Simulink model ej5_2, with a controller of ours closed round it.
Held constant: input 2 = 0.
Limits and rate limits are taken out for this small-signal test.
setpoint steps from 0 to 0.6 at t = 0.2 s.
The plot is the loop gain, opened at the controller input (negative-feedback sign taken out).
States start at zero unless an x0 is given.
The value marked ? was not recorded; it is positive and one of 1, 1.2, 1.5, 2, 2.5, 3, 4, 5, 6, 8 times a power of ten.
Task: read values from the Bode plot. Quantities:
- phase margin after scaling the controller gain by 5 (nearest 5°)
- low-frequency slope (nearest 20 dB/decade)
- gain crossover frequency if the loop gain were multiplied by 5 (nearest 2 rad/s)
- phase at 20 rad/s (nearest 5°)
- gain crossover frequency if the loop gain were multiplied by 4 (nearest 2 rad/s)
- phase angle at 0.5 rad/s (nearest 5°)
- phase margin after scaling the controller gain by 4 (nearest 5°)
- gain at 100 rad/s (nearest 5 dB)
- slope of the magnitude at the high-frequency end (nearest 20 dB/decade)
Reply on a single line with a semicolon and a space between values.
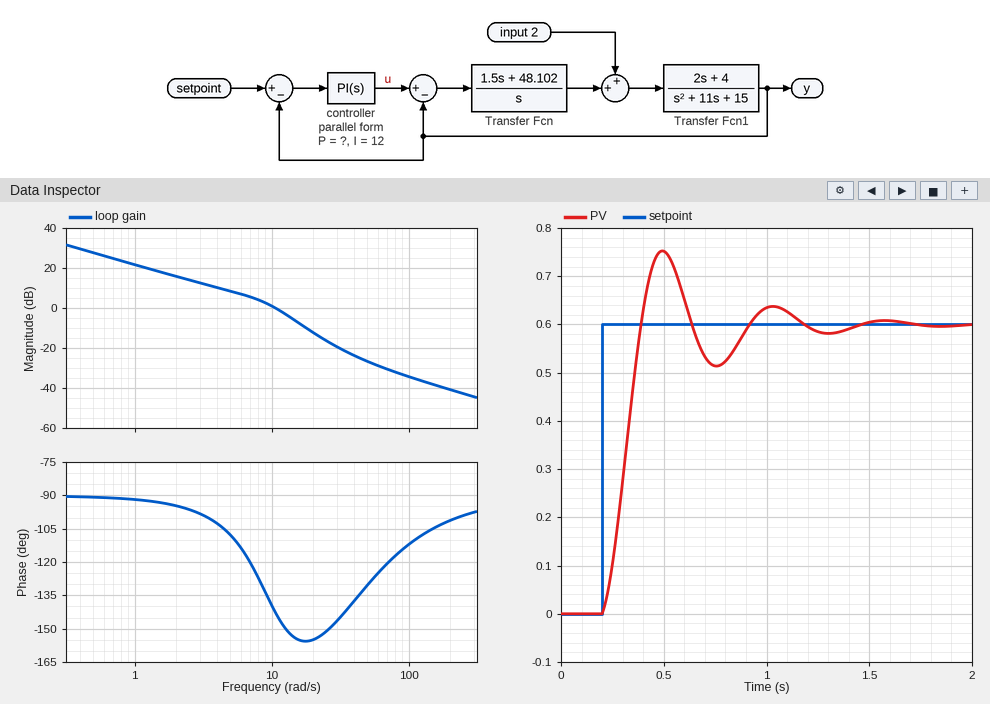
25°; -20 dB/decade; 22 rad/s; -155°; 20 rad/s; -90°; 25°; -35 dB; -20 dB/decade
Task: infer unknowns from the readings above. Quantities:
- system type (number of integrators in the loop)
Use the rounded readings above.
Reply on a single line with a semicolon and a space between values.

1
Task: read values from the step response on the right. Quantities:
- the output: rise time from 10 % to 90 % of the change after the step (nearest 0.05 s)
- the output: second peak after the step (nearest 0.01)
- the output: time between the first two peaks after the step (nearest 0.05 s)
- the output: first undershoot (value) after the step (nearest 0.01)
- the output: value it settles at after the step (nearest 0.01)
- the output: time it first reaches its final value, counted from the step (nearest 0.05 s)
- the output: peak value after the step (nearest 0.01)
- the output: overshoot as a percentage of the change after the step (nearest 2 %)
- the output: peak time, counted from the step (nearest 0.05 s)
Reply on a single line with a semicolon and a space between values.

0.15 s; 0.64; 0.55 s; 0.51; 0.60; 0.20 s; 0.75; 26 %; 0.30 s
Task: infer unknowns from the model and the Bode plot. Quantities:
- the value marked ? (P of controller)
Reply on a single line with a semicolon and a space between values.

0.6
